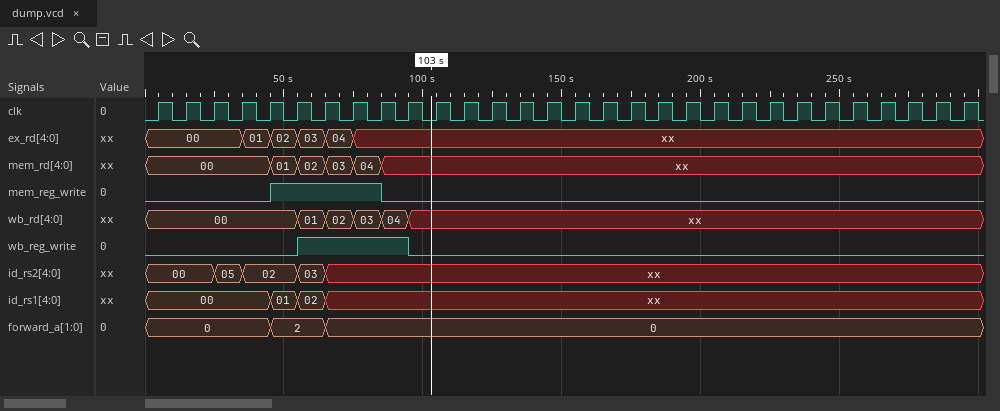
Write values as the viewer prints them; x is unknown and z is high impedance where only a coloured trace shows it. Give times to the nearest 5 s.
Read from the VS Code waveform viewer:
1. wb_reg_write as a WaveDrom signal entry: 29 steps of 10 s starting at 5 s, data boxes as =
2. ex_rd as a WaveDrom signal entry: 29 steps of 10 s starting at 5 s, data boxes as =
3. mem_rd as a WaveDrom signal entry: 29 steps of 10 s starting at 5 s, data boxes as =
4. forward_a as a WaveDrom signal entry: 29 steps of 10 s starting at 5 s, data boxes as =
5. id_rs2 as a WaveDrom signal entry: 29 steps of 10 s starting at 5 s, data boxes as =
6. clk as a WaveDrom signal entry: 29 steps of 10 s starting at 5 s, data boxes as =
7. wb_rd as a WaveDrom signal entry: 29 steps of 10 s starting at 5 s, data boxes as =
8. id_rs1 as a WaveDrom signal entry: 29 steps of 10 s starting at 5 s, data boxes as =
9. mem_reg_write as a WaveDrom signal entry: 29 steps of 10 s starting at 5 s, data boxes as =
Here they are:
{name: 'wb_reg_write', wave: '0....1...0...................'}
{name: 'ex_rd', wave: '=..====x.....................', data: '00 01 02 03 04'}
{name: 'mem_rd', wave: '=...====x....................', data: '00 01 02 03 04'}
{name: 'forward_a', wave: '=...=.=......................', data: '0 2 0'}
{name: 'id_rs2', wave: '=.==.=x......................', data: '00 05 02 03'}
{name: 'clk', wave: 'p............................'}
{name: 'wb_rd', wave: '=....====x...................', data: '00 01 02 03 04'}
{name: 'id_rs1', wave: '=...==x......................', data: '00 01 02'}
{name: 'mem_reg_write', wave: '0...1...0....................'}
